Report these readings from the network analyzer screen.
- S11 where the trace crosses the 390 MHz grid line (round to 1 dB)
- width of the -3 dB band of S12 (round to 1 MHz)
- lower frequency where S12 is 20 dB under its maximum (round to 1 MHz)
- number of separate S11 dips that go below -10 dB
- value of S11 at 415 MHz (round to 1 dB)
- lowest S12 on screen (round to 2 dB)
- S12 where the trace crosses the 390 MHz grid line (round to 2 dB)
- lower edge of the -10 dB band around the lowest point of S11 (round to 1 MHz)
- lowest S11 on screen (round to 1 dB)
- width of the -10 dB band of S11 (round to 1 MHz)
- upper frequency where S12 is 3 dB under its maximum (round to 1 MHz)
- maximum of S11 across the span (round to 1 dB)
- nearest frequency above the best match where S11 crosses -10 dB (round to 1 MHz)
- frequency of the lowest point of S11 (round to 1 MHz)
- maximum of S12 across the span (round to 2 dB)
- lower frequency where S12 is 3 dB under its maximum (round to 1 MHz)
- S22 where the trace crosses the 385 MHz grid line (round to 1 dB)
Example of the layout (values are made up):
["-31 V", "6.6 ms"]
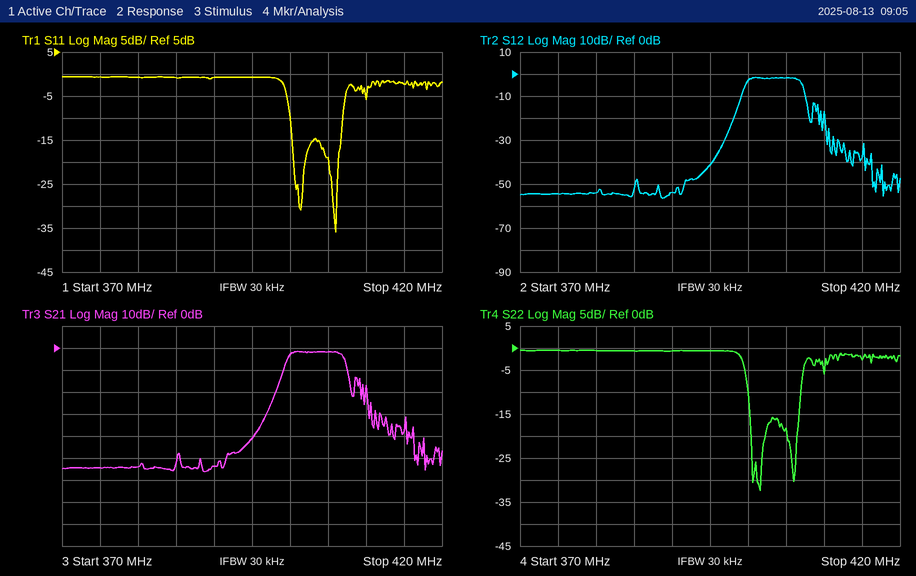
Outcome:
["-1 dB", "7 MHz", "398 MHz", "2", "-2 dB", "-56 dB", "-54 dB", "400 MHz", "-36 dB", "7 MHz", "407 MHz", "-1 dB", "407 MHz", "406 MHz", "-2 dB", "400 MHz", "-1 dB"]
